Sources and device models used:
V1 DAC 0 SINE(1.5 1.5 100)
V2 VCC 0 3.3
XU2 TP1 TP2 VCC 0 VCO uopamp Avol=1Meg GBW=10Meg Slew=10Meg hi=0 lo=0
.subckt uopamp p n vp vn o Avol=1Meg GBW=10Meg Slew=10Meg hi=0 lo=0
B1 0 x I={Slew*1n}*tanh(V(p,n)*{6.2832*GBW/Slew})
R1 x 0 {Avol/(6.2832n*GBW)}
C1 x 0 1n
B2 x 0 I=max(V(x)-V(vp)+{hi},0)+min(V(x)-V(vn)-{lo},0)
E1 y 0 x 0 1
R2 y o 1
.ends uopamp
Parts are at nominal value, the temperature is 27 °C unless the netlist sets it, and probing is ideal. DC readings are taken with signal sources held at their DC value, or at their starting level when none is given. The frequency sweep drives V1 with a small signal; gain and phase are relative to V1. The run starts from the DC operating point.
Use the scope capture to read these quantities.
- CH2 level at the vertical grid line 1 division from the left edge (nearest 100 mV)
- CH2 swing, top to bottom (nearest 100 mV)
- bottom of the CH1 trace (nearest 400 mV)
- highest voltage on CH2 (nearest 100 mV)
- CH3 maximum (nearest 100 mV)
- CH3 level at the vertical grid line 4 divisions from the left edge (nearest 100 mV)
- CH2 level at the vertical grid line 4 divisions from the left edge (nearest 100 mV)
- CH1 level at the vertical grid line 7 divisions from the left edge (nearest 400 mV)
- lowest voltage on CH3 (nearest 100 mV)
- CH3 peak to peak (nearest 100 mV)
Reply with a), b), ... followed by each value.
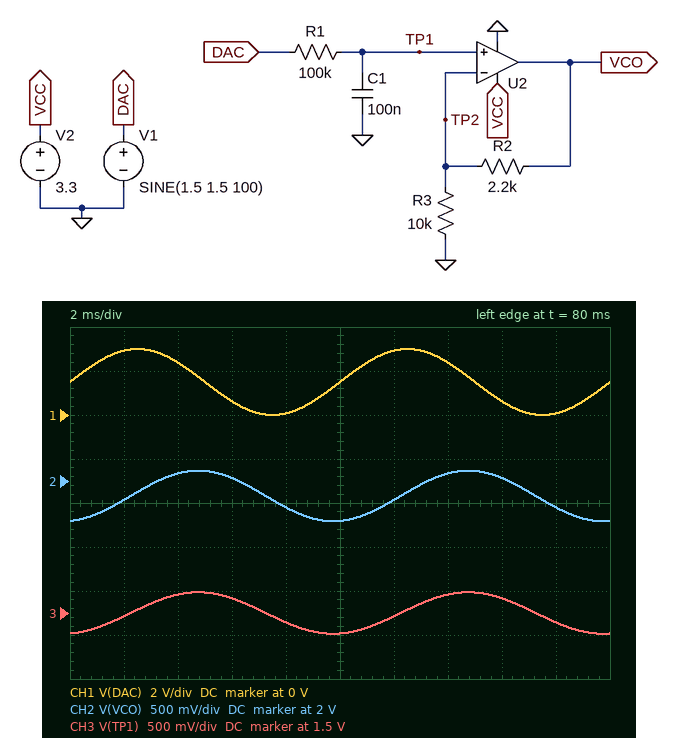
a) 1.8 V
b) 600 mV
c) 0 V
d) 2.1 V
e) 1.7 V
f) 1.4 V
g) 1.7 V
h) 2.4 V
i) 1.3 V
j) 500 mV
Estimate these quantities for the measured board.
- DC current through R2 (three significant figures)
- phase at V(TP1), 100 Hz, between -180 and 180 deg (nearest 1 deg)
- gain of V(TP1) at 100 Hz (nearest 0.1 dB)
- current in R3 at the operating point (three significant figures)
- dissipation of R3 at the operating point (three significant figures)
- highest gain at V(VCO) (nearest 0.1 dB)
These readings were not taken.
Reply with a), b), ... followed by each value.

a) 150 µA
b) -81 deg
c) -16.1 dB
d) 150 µA
e) 225 µW
f) 1.7 dB
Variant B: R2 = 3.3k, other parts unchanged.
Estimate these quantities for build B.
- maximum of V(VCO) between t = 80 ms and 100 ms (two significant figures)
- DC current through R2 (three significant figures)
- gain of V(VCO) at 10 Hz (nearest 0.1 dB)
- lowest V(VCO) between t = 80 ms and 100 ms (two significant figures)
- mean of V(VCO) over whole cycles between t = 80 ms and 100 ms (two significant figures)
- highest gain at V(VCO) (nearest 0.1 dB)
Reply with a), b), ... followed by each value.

a) 2.3 V
b) 150 µA
c) 1.0 dB
d) 1.7 V
e) 2.0 V
f) 2.5 dB
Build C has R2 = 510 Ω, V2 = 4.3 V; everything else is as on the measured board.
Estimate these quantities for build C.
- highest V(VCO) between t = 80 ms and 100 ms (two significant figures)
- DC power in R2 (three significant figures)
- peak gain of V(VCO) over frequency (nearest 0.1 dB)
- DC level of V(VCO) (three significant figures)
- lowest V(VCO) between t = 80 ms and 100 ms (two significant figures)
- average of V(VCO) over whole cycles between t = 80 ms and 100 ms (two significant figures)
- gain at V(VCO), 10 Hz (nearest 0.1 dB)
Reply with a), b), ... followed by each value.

a) 1.8 V
b) 11.5 µW
c) 0.4 dB
d) 1.58 V
e) 1.3 V
f) 1.6 V
g) -1.0 dB
